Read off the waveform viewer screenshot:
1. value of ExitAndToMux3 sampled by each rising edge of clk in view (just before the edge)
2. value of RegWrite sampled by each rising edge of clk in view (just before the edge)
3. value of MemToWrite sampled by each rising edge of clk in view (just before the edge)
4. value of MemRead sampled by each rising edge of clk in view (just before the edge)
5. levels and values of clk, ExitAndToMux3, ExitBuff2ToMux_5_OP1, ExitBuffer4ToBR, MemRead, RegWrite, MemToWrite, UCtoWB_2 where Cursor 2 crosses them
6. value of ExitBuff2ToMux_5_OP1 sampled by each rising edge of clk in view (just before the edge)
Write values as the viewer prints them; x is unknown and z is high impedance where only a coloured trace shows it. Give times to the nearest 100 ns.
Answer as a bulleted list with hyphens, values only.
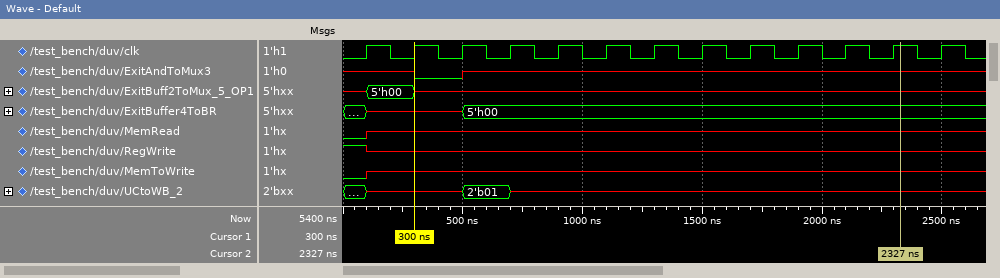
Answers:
- x x 0 x x x x x x x x x x
- 1 x x x x x x x x x x x x
- 0 x x x x x x x x x x x x
- 0 x x x x x x x x x x x x
- clk=1, ExitAndToMux3=x, ExitBuff2ToMux_5_OP1=x, ExitBuffer4ToBR=5'h00, MemRead=x, RegWrite=x, MemToWrite=x, UCtoWB_2=x
- x, 5'h00, x, x, x, x, x, x, x, x, x, x, x
